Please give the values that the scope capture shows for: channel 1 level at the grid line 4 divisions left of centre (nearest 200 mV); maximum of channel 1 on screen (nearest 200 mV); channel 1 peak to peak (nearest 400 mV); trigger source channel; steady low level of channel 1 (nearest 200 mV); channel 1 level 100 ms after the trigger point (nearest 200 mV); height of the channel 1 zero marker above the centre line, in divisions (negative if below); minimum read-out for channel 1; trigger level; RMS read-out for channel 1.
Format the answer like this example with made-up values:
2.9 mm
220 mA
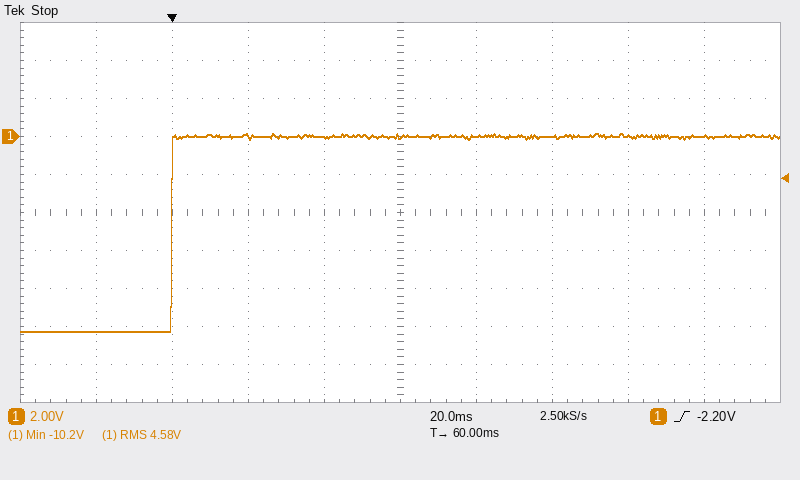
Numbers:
-10.2 V
200 mV
10.4 V
channel 1
-10.2 V
0.0 V
+2.0 div
-10.2 V
-2.20 V
4.58 V
